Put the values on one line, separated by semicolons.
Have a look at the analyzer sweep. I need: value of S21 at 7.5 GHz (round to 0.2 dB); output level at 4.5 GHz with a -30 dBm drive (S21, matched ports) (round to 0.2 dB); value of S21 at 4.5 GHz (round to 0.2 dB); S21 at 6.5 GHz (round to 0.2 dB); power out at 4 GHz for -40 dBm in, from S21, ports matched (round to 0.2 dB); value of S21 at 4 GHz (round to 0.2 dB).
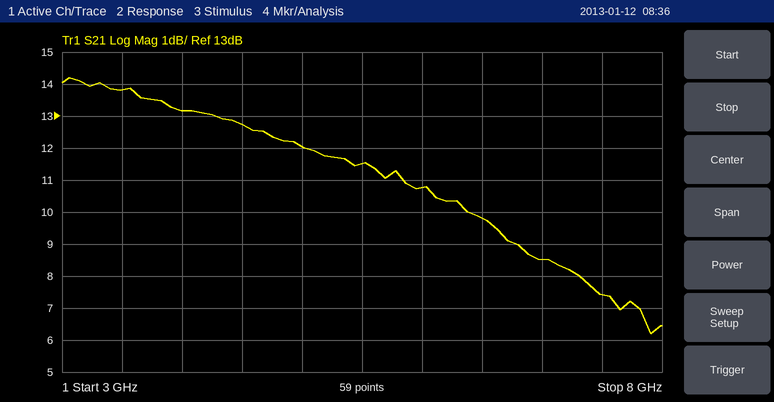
7.4 dB; -17.2 dBm; 12.8 dB; 9.8 dB; -26.8 dBm; 13.2 dB
